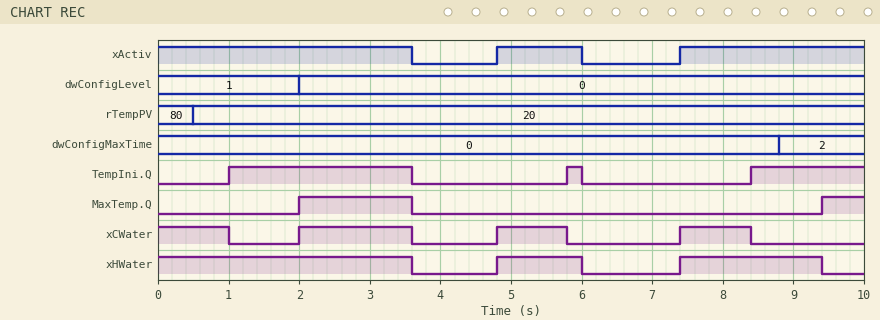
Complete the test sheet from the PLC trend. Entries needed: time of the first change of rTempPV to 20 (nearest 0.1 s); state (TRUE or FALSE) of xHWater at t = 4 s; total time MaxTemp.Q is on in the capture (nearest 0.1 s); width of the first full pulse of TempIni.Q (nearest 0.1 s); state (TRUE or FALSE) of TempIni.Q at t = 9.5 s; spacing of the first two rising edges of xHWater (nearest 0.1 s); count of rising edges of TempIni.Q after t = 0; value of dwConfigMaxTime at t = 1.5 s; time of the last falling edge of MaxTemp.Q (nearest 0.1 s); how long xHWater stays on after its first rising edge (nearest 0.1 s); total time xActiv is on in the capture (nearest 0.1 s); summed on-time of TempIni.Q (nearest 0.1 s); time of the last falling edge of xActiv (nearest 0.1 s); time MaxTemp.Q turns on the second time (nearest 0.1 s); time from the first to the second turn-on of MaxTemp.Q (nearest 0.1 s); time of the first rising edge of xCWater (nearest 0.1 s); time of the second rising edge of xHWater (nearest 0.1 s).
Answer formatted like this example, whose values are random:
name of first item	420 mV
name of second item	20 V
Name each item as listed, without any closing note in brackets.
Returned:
time of the first change of rTempPV to 20	0.5 s
state (TRUE or FALSE) of xHWater at t = 4 s	FALSE
total time MaxTemp.Q is on in the capture	2.2 s
width of the first full pulse of TempIni.Q	2.6 s
state (TRUE or FALSE) of TempIni.Q at t = 9.5 s	TRUE
spacing of the first two rising edges of xHWater	2.6 s
count of rising edges of TempIni.Q after t = 0	3
value of dwConfigMaxTime at t = 1.5 s	0
time of the last falling edge of MaxTemp.Q	3.6 s
how long xHWater stays on after its first rising edge	1.2 s
total time xActiv is on in the capture	7.4 s
summed on-time of TempIni.Q	4.4 s
time of the last falling edge of xActiv	6.0 s
time MaxTemp.Q turns on the second time	9.4 s
time from the first to the second turn-on of MaxTemp.Q	7.4 s
time of the first rising edge of xCWater	2.0 s
time of the second rising edge of xHWater	7.4 s
